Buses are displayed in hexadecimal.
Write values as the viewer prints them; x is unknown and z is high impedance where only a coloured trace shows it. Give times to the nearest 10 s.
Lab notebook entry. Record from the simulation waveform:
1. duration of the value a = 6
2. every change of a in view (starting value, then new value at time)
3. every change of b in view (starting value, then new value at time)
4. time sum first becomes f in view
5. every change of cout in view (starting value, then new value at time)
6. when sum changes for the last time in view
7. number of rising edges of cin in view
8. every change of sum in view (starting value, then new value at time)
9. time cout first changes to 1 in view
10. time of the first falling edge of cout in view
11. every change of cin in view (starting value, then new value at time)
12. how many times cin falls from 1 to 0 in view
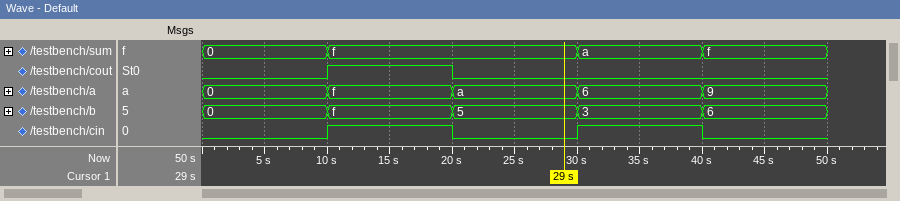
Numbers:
10 s
0, f at 10 s, a at 20 s, 6 at 30 s, 9 at 40 s
0, f at 10 s, 5 at 20 s, 3 at 30 s, 6 at 40 s
10 s
0, 1 at 10 s, 0 at 20 s
40 s
2
0, f at 10 s, a at 30 s, f at 40 s
10 s
20 s
0, 1 at 10 s, 0 at 20 s, 1 at 30 s, 0 at 40 s
2
